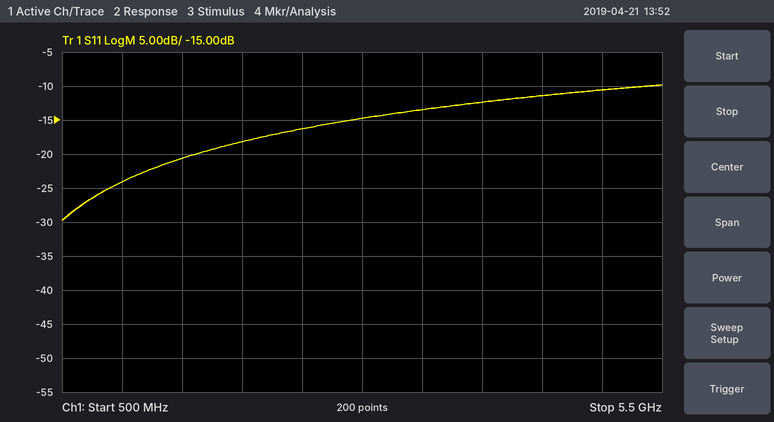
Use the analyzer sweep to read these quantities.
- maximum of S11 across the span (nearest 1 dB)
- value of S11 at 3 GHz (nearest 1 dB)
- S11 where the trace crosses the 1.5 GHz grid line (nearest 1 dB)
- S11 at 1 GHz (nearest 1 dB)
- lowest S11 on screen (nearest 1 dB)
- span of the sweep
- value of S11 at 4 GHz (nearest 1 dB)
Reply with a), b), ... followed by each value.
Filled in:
a) -10 dB
b) -15 dB
c) -21 dB
d) -24 dB
e) -30 dB
f) 5 GHz
g) -12 dB
